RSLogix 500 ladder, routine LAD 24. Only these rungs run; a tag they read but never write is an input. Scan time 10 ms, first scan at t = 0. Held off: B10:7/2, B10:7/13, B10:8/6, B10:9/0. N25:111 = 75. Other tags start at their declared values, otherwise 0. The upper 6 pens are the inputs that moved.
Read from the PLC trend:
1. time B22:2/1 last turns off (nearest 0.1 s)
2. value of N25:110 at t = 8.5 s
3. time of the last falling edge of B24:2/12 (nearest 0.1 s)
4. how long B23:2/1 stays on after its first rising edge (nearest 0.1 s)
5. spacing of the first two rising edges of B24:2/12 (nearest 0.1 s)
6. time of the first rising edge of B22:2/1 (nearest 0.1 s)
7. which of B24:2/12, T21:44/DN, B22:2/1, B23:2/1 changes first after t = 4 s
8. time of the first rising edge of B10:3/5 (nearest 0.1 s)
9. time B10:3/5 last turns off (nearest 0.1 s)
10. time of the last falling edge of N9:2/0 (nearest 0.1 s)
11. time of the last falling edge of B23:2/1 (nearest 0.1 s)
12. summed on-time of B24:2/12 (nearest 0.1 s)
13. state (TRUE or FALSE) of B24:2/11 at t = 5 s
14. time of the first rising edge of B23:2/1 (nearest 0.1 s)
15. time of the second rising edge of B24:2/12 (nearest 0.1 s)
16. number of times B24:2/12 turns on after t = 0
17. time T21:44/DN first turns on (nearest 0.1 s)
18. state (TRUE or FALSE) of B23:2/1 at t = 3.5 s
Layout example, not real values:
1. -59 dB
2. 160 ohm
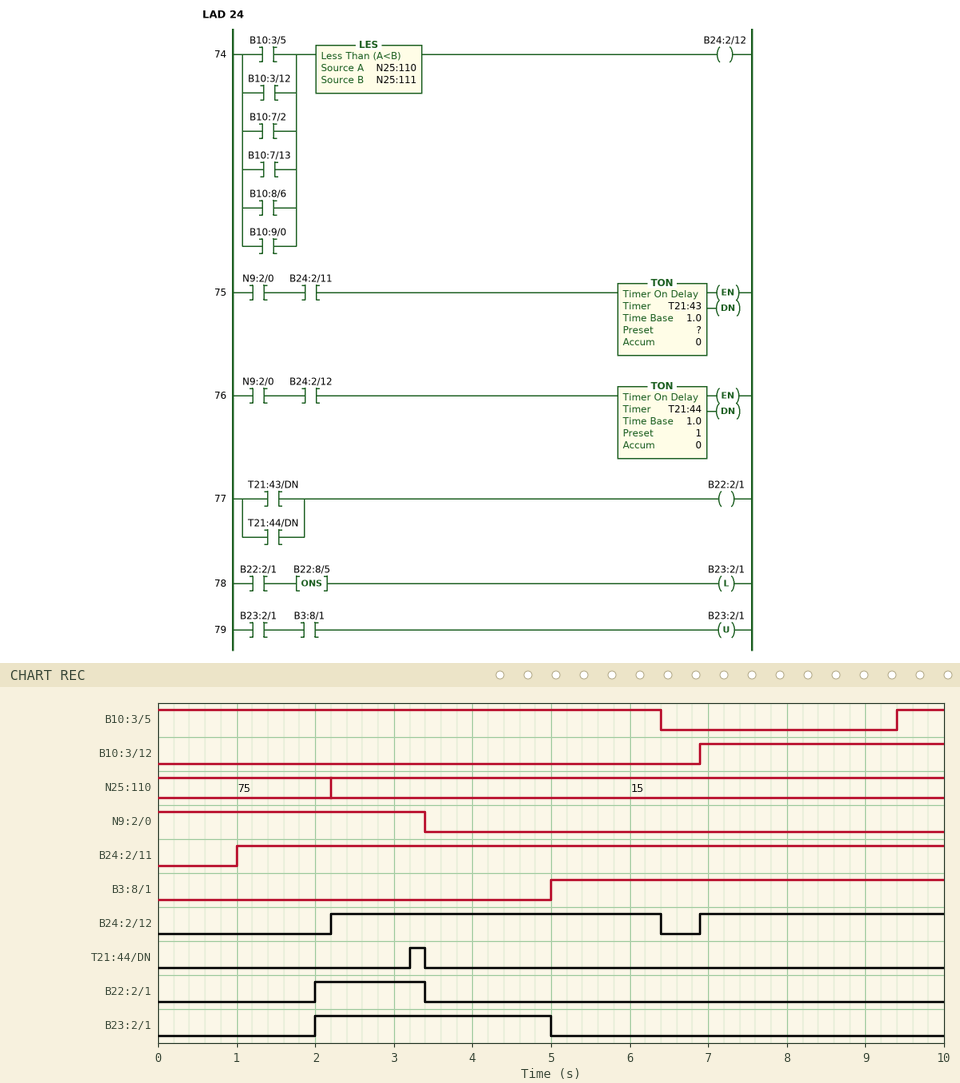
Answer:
1. 3.4 s
2. 15
3. 6.4 s
4. 3.0 s
5. 4.7 s
6. 2.0 s
7. B23:2/1
8. 9.4 s
9. 6.4 s
10. 3.4 s
11. 5.0 s
12. 7.3 s
13. TRUE
14. 2.0 s
15. 6.9 s
16. 2
17. 3.2 s
18. TRUE
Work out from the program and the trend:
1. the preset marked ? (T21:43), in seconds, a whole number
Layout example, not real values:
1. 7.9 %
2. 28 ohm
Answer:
1. 1 s
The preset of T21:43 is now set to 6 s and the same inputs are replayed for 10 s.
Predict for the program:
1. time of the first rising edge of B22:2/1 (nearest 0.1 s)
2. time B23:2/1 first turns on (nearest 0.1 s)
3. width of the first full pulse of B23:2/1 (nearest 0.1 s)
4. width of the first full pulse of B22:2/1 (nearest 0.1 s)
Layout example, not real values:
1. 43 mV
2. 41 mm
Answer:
1. 3.2 s
2. 3.2 s
3. 1.8 s
4. 0.2 s
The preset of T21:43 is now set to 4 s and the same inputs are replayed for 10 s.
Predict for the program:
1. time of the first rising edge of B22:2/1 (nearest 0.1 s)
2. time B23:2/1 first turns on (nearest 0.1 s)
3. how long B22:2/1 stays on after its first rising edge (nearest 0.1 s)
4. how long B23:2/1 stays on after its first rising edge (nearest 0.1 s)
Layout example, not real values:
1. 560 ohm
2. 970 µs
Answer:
1. 3.2 s
2. 3.2 s
3. 0.2 s
4. 1.8 s
